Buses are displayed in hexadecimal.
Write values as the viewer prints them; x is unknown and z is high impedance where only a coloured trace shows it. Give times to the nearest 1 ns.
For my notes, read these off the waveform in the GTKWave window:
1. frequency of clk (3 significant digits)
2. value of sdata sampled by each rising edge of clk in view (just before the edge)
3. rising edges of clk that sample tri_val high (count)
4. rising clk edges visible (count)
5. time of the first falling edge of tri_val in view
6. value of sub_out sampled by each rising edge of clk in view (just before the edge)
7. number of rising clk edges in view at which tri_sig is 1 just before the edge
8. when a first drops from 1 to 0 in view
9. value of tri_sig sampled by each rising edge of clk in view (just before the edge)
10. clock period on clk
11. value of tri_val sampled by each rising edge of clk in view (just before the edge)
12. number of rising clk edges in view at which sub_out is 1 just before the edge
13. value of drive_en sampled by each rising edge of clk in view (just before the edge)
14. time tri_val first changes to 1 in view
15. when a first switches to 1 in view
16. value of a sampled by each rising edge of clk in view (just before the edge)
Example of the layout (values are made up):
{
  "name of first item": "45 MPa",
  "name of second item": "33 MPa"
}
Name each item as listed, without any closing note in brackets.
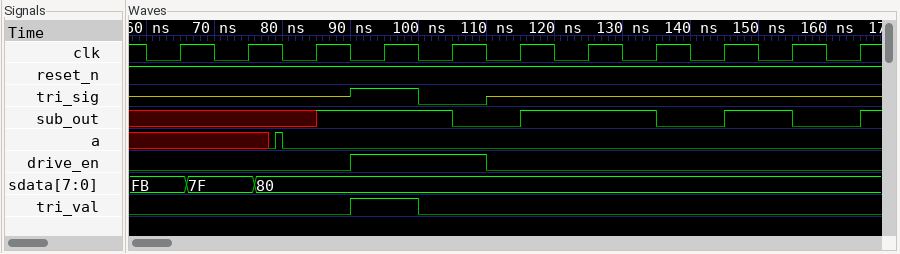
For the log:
{
  "frequency of clk": "100 MHz",
  "value of sdata sampled by each rising edge of clk in view": "FB, 7F, 80, 80, 80, 80, 80, 80, 80, 80, 80",
  "rising edges of clk that sample tri_val high": "1",
  "rising clk edges visible": "11",
  "time of the first falling edge of tri_val in view": "100 ns",
  "value of sub_out sampled by each rising edge of clk in view": "x x x 1 1 0 1 1 0 1 0",
  "number of rising clk edges in view at which tri_sig is 1 just before the edge": "1",
  "when a first drops from 1 to 0 in view": "80 ns",
  "value of tri_sig sampled by each rising edge of clk in view": "z z z 1 0 z z z z z z",
  "clock period on clk": "10 ns",
  "value of tri_val sampled by each rising edge of clk in view": "0 0 0 1 0 0 0 0 0 0 0",
  "number of rising clk edges in view at which sub_out is 1 just before the edge": "5",
  "value of drive_en sampled by each rising edge of clk in view": "0 0 0 1 1 0 0 0 0 0 0",
  "time tri_val first changes to 1 in view": "90 ns",
  "when a first switches to 1 in view": "79 ns",
  "value of a sampled by each rising edge of clk in view": "x x 0 0 0 0 0 0 0 0 0"
}
